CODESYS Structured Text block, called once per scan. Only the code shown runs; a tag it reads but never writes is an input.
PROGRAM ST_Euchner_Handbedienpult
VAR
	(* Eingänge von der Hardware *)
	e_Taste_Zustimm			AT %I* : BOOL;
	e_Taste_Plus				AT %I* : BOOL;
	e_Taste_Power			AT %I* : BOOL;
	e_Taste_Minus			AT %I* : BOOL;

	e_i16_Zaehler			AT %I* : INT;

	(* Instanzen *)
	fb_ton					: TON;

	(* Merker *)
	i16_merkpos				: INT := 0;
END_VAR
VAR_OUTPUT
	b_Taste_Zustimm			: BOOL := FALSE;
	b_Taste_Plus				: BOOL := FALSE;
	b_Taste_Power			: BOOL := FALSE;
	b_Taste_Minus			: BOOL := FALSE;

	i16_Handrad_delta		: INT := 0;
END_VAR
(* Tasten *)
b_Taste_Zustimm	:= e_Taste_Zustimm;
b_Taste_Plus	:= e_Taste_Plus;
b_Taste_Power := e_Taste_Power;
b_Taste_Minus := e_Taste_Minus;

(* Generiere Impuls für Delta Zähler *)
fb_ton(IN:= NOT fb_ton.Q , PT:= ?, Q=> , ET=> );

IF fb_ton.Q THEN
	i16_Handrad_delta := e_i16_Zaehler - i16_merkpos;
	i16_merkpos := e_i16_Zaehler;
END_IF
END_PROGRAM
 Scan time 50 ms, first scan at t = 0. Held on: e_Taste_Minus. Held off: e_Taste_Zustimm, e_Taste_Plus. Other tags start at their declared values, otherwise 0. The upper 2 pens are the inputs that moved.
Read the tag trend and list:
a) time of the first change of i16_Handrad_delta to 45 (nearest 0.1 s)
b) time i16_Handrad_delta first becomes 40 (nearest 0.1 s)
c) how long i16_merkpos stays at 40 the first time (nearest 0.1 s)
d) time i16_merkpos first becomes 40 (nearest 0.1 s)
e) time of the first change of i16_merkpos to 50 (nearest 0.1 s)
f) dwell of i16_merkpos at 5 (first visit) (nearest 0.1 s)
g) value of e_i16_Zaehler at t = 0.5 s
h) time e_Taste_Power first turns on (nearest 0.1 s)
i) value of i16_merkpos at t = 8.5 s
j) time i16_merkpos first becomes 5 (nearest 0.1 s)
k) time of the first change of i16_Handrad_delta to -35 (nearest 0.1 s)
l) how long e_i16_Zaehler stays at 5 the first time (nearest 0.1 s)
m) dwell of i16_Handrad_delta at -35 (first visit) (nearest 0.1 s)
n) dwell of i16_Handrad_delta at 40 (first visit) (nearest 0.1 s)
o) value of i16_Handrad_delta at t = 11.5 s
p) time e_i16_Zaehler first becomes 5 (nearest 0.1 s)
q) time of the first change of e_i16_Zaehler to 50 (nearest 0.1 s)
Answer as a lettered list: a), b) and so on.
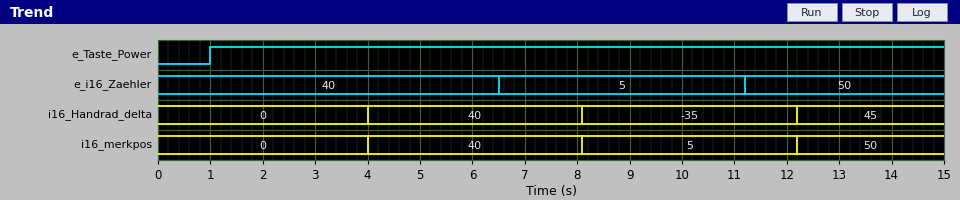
a) 12.2 s
b) 4.0 s
c) 4.1 s
d) 4.0 s
e) 12.2 s
f) 4.1 s
g) 40
h) 1.0 s
i) 5
j) 8.1 s
k) 8.1 s
l) 4.7 s
m) 4.1 s
n) 4.1 s
o) -35
p) 6.5 s
q) 11.2 s
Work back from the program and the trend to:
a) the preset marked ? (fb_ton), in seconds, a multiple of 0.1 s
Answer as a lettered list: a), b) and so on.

a) 4.0 s
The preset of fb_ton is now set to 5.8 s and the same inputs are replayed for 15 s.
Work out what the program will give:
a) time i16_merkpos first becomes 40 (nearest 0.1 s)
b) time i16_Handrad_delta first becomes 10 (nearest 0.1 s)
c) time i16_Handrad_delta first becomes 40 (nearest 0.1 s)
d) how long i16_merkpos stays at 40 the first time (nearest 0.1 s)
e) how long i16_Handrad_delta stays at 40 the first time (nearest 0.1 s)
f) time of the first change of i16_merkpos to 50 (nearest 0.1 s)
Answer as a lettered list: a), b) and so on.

a) 5.8 s
b) 11.7 s
c) 5.8 s
d) 5.9 s
e) 5.9 s
f) 11.7 s
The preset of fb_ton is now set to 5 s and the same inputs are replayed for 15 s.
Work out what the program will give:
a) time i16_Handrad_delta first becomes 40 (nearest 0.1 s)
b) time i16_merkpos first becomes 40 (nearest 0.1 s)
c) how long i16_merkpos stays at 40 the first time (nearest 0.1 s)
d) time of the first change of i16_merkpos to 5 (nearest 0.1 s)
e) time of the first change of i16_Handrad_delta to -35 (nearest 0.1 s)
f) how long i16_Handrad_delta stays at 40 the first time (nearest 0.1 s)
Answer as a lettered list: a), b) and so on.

a) 5.0 s
b) 5.0 s
c) 5.1 s
d) 10.1 s
e) 10.1 s
f) 5.1 s
